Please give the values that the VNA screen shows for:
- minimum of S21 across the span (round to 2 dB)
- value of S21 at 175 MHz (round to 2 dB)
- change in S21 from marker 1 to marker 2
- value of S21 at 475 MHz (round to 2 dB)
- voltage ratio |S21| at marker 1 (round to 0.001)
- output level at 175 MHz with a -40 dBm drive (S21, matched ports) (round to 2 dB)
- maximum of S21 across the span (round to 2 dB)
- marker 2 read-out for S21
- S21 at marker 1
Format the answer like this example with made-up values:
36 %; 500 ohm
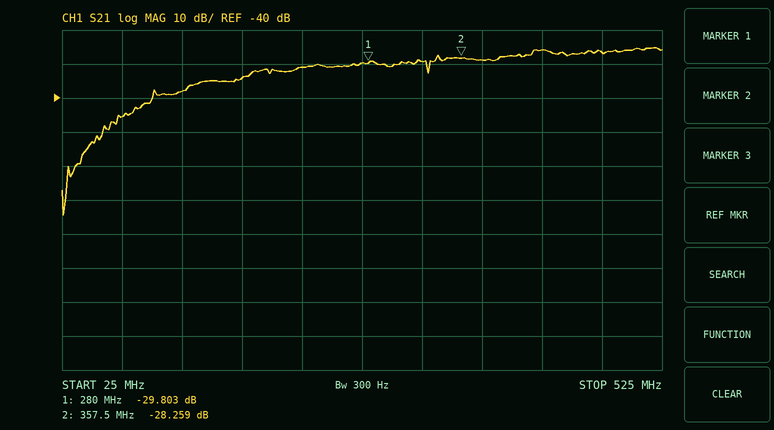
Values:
-74 dB; -34 dB; 1.544 dB; -26 dB; 0.032; -74 dBm; -26 dB; -28.259 dB; -29.803 dB
